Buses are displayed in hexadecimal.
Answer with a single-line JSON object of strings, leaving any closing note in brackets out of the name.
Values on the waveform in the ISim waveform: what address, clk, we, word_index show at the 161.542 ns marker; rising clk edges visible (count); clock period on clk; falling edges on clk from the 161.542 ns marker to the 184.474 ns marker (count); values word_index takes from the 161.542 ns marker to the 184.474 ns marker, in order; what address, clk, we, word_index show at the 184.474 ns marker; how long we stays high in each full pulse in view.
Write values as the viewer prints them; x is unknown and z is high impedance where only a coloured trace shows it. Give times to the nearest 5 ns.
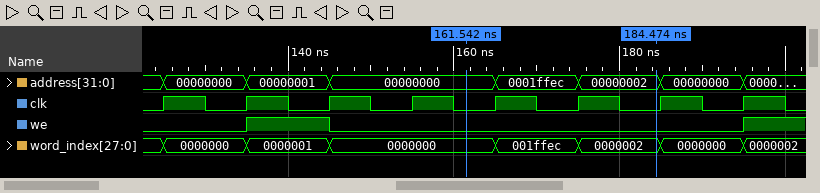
{"what address, clk, we, word_index show at the 161.542 ns marker": "address=00000000, clk=0, we=0, word_index=0000000", "rising clk edges visible": "8", "clock period on clk": "10 ns", "falling edges on clk from the 161.542 ns marker to the 184.474 ns marker": "2", "values word_index takes from the 161.542 ns marker to the 184.474 ns marker, in order": "0000000, 001ffec, 0000002", "what address, clk, we, word_index show at the 184.474 ns marker": "address=00000002, clk=0, we=0, word_index=0000002", "how long we stays high in each full pulse in view": "10 ns"}
